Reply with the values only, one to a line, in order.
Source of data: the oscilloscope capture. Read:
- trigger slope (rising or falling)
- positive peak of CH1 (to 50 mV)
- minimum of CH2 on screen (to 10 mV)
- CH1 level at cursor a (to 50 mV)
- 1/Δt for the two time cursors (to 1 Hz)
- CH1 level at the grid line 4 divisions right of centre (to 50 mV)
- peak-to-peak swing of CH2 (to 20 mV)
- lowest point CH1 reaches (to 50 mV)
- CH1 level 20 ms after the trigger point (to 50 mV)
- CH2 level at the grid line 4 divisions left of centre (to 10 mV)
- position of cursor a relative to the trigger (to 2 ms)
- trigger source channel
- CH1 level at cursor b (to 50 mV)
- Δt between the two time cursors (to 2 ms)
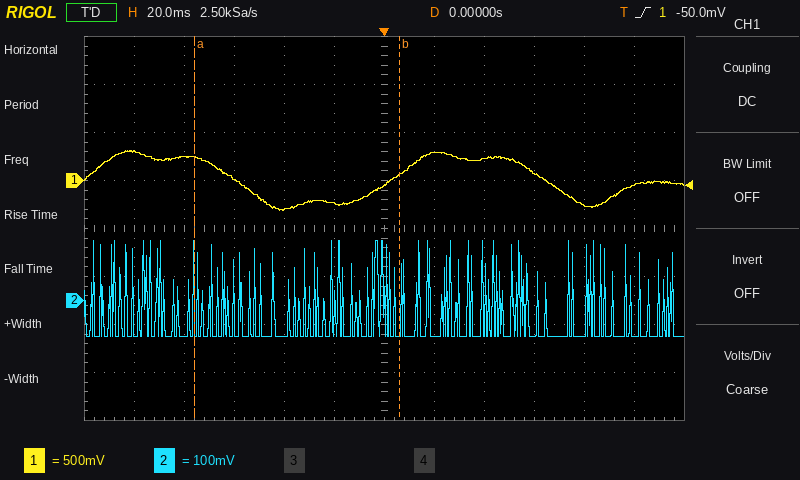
rising
300 mV
-80 mV
250 mV
12 Hz
-250 mV
200 mV
-300 mV
300 mV
-80 mV
-76 ms
CH1
50 mV
82 ms
